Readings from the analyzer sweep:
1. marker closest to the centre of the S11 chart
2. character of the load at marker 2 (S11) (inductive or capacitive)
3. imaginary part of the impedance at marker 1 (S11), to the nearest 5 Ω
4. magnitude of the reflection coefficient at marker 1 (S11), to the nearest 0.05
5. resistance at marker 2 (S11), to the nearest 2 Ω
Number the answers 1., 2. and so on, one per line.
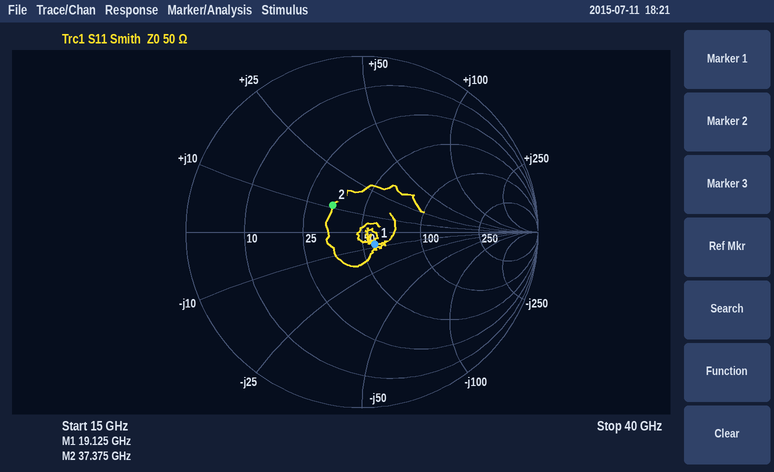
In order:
1. marker 1
2. inductive
3. -10 Ω
4. 0.10
5. 34 Ω
